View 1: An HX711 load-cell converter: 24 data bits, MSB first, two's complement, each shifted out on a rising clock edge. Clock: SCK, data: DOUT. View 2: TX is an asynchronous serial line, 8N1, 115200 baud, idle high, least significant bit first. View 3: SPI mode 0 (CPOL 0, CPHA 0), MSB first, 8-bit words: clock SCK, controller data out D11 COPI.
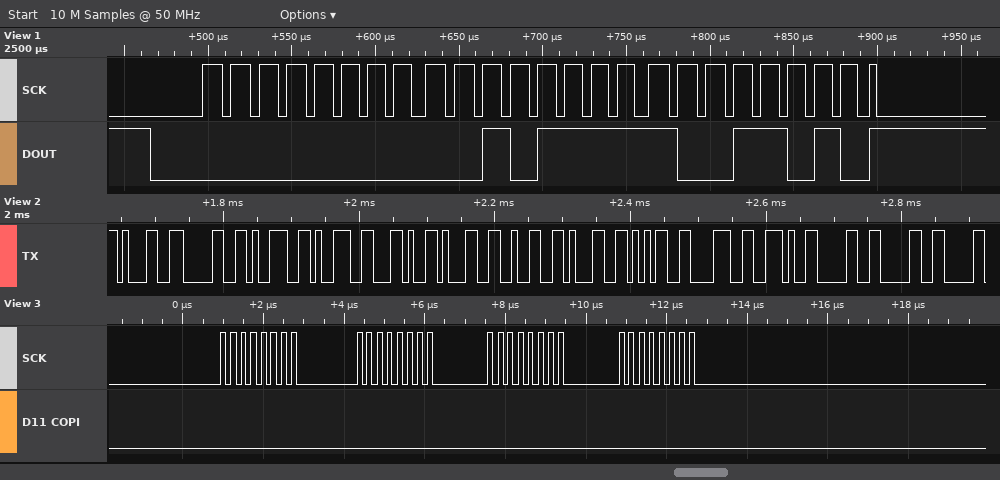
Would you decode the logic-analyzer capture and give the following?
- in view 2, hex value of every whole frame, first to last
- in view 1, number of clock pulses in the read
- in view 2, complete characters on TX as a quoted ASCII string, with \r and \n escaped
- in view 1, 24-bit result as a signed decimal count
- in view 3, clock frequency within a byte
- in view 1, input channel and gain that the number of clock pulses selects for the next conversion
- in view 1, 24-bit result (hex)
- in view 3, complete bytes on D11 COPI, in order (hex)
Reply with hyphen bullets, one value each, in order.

- 0x31 0x30 0x39 0x39 0x2C 0x31 0x32 0x31 0x35 0x38 0x2E 0x30 0x30
- 25
- "1099,12158.00"
- 12186
- 4 MHz
- channel A, gain 128
- 0x002F9A
- 00 00 00 00
